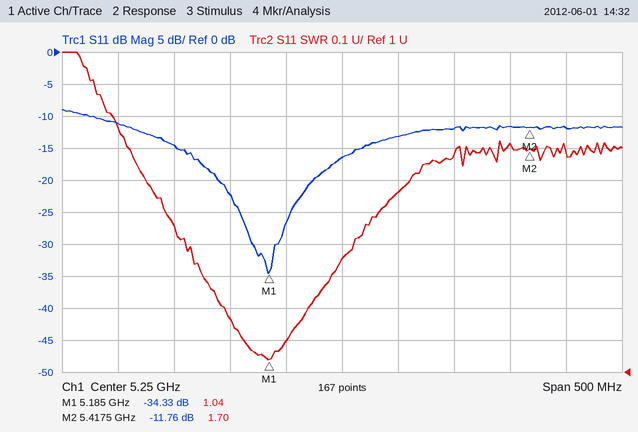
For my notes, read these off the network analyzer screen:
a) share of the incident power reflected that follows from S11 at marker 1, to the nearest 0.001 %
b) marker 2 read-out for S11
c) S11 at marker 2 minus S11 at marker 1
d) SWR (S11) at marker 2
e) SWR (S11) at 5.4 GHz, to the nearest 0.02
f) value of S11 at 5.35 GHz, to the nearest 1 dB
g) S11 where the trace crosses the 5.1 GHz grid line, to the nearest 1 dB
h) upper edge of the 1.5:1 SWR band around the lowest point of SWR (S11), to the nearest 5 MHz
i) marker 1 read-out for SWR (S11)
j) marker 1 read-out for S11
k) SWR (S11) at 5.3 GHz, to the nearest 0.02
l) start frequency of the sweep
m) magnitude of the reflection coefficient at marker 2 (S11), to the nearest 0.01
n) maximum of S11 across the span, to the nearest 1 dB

0.037 %
-11.76 dB
22.57 dB
1.70
1.72
-12 dB
-15 dB
5.285 GHz
1.04
-34.33 dB
1.56
5 GHz
0.26
-9 dB
